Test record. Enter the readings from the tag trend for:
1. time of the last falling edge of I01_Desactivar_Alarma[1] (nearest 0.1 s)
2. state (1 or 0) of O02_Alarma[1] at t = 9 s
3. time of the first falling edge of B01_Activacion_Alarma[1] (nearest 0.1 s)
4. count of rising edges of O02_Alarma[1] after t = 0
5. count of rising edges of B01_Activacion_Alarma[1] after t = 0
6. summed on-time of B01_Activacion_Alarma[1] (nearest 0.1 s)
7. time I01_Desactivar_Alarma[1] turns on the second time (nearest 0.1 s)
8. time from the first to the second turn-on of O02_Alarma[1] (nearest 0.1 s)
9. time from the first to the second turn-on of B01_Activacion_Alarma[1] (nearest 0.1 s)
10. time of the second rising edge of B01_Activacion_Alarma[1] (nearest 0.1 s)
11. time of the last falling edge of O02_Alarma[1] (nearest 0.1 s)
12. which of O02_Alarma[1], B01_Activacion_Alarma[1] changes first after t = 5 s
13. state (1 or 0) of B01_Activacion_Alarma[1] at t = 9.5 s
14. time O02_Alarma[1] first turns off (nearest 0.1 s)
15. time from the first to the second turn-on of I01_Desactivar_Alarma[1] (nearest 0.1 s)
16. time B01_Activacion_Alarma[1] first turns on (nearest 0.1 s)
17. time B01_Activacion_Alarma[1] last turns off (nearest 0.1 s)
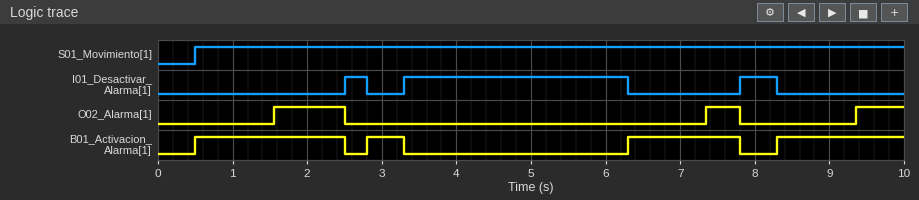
8.3 s
0
2.5 s
3
4
5.7 s
3.3 s
5.8 s
2.3 s
2.8 s
7.8 s
B01_Activacion_Alarma[1]
1
2.5 s
0.8 s
0.5 s
7.8 s
